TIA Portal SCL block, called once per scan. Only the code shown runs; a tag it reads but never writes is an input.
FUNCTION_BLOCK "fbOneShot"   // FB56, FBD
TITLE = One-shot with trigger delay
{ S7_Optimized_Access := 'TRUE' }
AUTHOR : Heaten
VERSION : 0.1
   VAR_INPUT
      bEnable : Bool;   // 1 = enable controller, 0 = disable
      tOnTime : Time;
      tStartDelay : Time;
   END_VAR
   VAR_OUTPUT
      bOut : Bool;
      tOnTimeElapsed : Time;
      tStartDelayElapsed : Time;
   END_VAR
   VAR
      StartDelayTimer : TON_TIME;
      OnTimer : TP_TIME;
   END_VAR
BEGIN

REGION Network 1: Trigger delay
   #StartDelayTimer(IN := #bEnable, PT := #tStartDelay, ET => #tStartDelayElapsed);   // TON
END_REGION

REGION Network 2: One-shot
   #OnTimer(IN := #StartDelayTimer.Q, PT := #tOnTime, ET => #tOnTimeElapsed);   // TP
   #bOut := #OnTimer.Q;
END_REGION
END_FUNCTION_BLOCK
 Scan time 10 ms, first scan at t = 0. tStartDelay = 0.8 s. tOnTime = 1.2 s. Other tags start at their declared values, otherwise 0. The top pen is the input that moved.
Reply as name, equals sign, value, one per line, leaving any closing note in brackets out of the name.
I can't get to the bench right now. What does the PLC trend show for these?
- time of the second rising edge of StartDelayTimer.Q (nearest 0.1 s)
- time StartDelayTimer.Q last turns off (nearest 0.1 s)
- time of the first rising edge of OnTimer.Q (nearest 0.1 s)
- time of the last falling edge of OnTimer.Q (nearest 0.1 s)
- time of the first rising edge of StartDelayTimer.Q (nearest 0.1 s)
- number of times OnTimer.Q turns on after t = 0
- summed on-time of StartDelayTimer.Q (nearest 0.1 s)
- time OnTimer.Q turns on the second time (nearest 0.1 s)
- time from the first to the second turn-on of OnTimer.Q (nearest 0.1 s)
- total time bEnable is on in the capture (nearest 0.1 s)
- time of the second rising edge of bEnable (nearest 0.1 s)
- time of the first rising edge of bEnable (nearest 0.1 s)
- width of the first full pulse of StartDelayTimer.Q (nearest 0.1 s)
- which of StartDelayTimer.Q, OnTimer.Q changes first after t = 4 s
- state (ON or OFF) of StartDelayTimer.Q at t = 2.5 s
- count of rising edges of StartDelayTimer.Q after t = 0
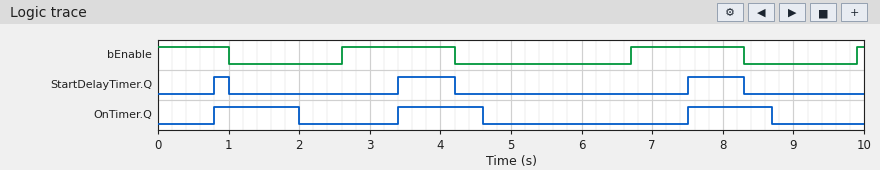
time of the second rising edge of StartDelayTimer.Q = 3.4 s
time StartDelayTimer.Q last turns off = 8.3 s
time of the first rising edge of OnTimer.Q = 0.8 s
time of the last falling edge of OnTimer.Q = 8.7 s
time of the first rising edge of StartDelayTimer.Q = 0.8 s
number of times OnTimer.Q turns on after t = 0 = 3
summed on-time of StartDelayTimer.Q = 1.8 s
time OnTimer.Q turns on the second time = 3.4 s
time from the first to the second turn-on of OnTimer.Q = 2.6 s
total time bEnable is on in the capture = 4.3 s
time of the second rising edge of bEnable = 6.7 s
time of the first rising edge of bEnable = 2.6 s
width of the first full pulse of StartDelayTimer.Q = 0.2 s
which of StartDelayTimer.Q, OnTimer.Q changes first after t = 4 s = StartDelayTimer.Q
state (ON or OFF) of StartDelayTimer.Q at t = 2.5 s = OFF
count of rising edges of StartDelayTimer.Q after t = 0 = 3
